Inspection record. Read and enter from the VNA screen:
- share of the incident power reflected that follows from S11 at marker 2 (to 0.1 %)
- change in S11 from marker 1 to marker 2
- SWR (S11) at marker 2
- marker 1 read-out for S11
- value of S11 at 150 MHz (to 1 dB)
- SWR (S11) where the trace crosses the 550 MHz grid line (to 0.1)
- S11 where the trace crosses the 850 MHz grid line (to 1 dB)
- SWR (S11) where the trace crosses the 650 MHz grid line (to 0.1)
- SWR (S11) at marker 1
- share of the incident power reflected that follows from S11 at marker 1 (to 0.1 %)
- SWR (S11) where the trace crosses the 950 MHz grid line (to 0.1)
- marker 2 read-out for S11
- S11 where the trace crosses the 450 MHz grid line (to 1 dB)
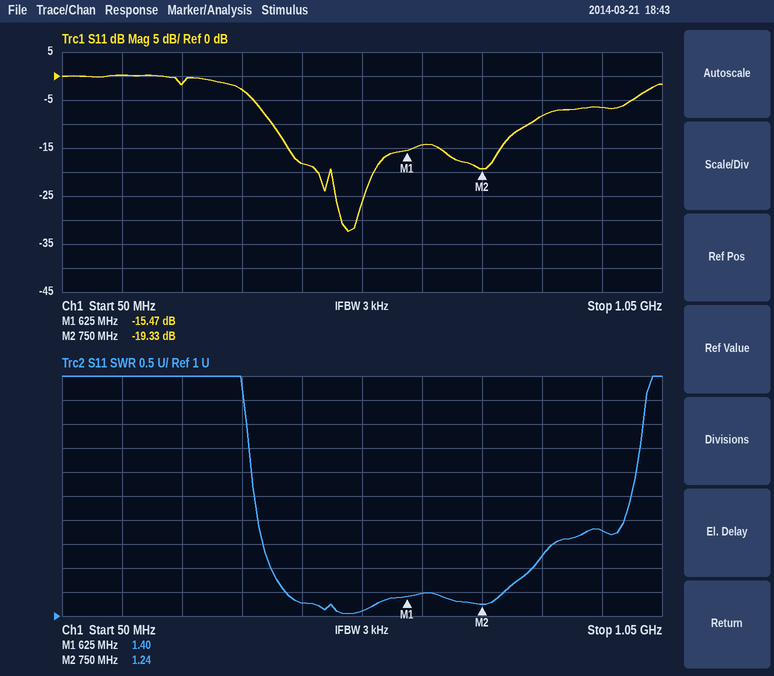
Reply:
1.2 %
-3.86 dB
1.24
-15.47 dB
0 dB
1.1
-8 dB
1.5
1.40
2.8 %
2.8
-19.33 dB
-18 dB
